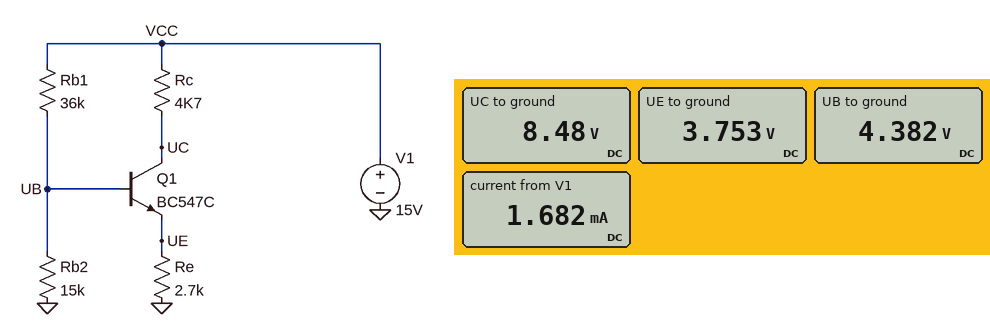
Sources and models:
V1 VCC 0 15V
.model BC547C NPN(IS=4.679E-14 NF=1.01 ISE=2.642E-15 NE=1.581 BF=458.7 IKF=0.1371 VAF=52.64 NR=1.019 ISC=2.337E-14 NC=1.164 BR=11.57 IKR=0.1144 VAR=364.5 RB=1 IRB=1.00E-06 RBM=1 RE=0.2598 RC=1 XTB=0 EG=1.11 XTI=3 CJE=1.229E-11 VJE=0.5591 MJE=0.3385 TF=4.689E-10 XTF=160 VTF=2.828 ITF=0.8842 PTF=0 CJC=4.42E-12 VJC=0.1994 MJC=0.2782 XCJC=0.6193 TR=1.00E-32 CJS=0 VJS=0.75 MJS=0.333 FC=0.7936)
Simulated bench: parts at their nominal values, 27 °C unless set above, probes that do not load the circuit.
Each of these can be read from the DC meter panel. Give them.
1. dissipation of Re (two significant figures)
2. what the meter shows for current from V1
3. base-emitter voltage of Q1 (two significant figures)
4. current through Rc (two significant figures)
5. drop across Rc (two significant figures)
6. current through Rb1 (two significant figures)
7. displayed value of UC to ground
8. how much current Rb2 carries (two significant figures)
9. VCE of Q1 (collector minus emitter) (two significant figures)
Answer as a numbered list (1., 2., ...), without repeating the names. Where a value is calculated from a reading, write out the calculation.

1. (3.753 V)^2 / 2.7 kΩ = 5.2 mW
2. 1.682 mA
3. 4.382 V - 3.753 V = 630 mV
4. (15 V - 8.48 V) / 4.7 kΩ = 1.4 mA
5. 15 V - 8.48 V = 6.5 V
6. (15 V - 4.382 V) / 36 kΩ = 290 µA
7. 8.48 V
8. (4.382 V) / 15 kΩ = 290 µA
9. 8.48 V - 3.753 V = 4.7 V
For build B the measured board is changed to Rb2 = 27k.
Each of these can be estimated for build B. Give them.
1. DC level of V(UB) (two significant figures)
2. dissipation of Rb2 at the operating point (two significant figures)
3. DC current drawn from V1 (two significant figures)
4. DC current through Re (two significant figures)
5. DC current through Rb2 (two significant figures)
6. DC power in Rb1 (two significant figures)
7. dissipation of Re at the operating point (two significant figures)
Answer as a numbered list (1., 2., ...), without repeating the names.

1. 6.1 V
2. 1.4 mW
3. 2.3 mA
4. 2.0 mA
5. 230 µA
6. 2.2 mW
7. 11 mW
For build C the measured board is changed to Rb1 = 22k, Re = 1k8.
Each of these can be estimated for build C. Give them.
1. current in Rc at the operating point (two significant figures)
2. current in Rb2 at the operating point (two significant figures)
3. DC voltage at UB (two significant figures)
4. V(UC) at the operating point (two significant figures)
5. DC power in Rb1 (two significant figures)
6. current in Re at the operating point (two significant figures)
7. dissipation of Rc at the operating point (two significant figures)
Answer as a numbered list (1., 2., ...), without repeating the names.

1. 2.3 mA
2. 330 µA
3. 5.0 V
4. 4.3 V
5. 4.6 mW
6. 2.4 mA
7. 24 mW
